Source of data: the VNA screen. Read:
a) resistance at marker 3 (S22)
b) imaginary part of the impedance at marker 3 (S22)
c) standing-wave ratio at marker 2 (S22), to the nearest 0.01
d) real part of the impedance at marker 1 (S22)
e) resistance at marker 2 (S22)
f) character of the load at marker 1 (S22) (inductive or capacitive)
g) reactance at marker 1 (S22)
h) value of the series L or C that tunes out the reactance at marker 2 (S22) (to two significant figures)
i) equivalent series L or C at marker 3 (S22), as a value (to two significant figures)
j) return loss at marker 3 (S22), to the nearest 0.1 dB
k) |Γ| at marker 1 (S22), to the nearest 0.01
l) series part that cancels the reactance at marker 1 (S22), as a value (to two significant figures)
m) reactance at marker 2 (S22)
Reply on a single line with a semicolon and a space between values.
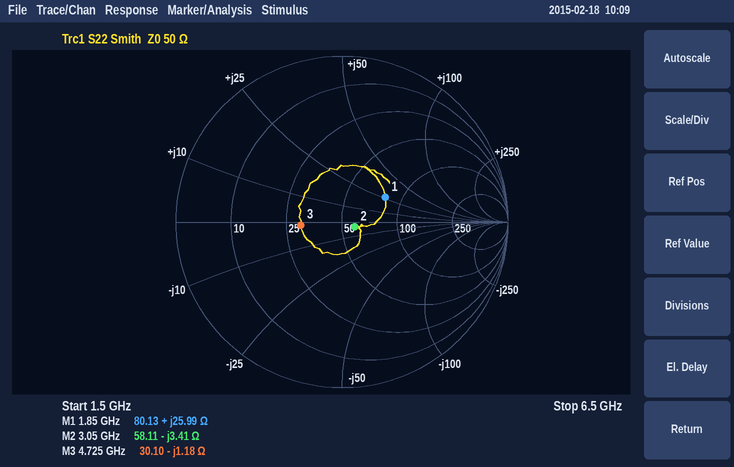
30.10 Ω; -1.18 Ω; 1.18; 80.13 Ω; 58.11 Ω; inductive; +25.99 Ω; 180 pH; 29 pF; 12.1 dB; 0.30; 3.3 pF; -3.41 Ω
